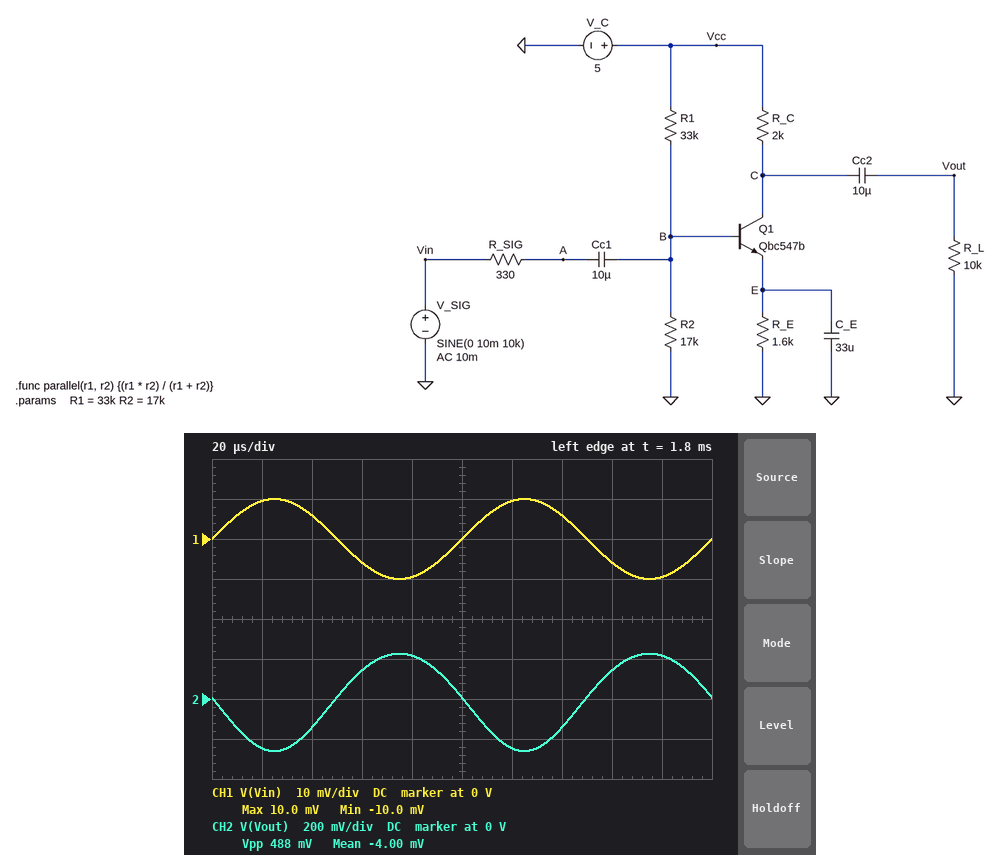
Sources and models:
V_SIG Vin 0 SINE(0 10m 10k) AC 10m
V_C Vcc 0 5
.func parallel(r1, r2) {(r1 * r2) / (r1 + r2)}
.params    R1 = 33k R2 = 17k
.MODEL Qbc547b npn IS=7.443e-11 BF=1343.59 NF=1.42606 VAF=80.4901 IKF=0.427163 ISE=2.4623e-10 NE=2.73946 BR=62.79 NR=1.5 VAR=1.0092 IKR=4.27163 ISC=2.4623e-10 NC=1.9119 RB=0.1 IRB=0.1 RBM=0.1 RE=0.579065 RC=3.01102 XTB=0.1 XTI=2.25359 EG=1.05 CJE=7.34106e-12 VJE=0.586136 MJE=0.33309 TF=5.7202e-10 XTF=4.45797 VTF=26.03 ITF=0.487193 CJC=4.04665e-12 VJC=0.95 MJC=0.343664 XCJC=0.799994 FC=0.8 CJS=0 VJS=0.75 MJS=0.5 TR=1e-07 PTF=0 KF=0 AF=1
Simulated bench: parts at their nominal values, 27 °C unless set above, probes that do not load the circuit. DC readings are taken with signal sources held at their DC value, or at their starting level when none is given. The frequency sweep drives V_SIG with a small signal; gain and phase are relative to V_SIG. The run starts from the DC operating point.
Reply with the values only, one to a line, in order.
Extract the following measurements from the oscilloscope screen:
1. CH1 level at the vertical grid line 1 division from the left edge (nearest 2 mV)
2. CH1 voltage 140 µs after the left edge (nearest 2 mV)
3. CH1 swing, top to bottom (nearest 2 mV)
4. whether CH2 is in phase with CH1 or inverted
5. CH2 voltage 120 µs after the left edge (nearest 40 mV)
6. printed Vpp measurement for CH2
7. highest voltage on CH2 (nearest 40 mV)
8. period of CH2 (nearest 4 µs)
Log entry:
10 mV
6 mV
20 mV
inverted
-240 mV
488 mV
240 mV
100 µs
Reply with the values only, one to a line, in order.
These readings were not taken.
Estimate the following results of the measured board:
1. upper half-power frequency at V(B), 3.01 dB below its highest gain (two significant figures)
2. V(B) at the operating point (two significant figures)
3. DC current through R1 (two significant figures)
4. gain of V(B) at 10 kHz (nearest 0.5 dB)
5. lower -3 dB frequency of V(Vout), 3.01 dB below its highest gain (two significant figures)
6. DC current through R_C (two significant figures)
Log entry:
4.6 MHz
1.7 V
100 µA
-0.5 dB
77 Hz
650 µA
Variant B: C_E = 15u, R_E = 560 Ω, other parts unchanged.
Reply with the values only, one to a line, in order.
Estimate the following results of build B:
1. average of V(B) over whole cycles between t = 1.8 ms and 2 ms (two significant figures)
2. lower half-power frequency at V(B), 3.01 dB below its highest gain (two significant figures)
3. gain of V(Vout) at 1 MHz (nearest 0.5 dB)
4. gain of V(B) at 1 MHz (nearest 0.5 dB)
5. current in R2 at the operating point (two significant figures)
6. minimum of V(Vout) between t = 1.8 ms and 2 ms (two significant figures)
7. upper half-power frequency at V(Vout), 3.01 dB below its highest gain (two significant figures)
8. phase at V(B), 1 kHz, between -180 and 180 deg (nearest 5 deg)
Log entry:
1.6 V
1.5 Hz
33.5 dB
-2.0 dB
96 µA
-450 mV
1.7 MHz
0 deg
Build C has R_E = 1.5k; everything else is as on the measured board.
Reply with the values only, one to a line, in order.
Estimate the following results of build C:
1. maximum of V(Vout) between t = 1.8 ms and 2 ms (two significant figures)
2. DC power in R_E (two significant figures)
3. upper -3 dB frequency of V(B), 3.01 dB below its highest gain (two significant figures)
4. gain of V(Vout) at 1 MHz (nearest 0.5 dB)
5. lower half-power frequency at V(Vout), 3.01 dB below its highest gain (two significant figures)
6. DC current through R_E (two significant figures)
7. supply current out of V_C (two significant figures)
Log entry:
240 mV
720 µW
4.4 MHz
28.0 dB
81 Hz
690 µA
790 µA
